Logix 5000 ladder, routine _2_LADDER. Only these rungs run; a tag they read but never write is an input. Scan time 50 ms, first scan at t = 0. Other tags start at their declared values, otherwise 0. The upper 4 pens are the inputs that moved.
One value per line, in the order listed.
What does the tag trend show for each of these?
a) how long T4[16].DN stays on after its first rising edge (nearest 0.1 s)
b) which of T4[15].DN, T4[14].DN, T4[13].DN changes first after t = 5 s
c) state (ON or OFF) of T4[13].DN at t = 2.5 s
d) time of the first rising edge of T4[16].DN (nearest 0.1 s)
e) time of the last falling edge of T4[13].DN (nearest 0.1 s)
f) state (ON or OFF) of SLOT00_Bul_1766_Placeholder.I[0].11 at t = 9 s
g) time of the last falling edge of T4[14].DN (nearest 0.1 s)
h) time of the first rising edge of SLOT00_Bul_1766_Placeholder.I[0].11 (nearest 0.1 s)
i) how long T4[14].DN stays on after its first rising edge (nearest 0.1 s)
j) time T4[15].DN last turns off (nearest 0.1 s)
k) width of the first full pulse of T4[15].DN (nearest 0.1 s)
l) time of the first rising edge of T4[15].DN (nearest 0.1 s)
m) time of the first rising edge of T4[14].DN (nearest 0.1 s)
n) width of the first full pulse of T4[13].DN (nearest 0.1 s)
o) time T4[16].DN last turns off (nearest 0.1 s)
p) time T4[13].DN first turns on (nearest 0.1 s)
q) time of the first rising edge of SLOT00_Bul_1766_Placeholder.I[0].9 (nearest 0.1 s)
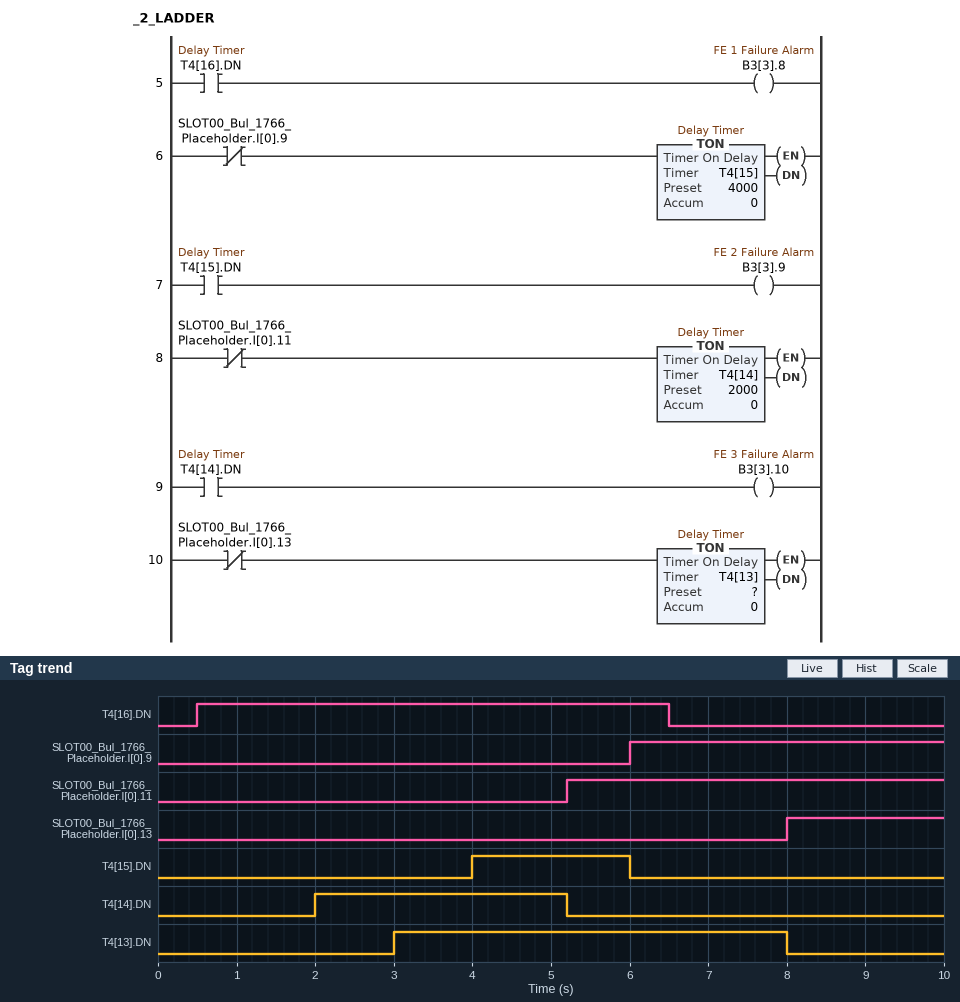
6.0 s
T4[14].DN
OFF
0.5 s
8.0 s
ON
5.2 s
5.2 s
3.2 s
6.0 s
2.0 s
4.0 s
2.0 s
5.0 s
6.5 s
3.0 s
6.0 s
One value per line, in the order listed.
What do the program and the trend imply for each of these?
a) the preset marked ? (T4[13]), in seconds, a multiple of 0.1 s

3.0 s
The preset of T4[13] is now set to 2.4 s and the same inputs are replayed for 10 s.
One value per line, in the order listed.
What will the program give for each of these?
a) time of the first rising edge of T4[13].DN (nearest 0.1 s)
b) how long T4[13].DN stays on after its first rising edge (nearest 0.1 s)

2.4 s
5.6 s
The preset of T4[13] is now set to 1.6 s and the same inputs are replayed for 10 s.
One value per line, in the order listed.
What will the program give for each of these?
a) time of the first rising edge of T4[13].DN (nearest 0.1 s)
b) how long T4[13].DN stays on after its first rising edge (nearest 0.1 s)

1.6 s
6.4 s
